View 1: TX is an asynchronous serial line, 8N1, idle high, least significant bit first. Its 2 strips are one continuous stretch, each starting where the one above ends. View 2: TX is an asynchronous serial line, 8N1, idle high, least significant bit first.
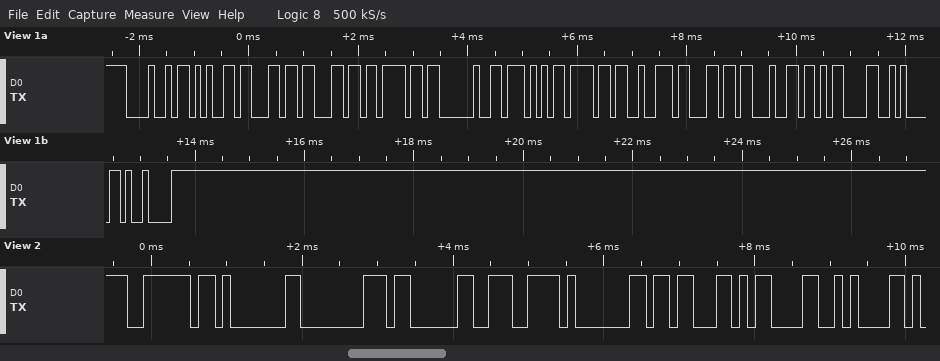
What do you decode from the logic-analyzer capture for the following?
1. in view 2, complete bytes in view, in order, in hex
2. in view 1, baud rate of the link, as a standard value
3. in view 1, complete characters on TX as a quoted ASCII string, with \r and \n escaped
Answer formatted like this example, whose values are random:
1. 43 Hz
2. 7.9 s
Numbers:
1. 7E 01 80 03 CE 01 1B 0D 0A
2. 9600 baud
3. "Hello World\r\n\t"
